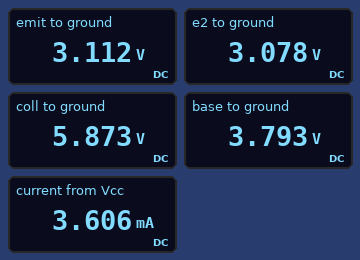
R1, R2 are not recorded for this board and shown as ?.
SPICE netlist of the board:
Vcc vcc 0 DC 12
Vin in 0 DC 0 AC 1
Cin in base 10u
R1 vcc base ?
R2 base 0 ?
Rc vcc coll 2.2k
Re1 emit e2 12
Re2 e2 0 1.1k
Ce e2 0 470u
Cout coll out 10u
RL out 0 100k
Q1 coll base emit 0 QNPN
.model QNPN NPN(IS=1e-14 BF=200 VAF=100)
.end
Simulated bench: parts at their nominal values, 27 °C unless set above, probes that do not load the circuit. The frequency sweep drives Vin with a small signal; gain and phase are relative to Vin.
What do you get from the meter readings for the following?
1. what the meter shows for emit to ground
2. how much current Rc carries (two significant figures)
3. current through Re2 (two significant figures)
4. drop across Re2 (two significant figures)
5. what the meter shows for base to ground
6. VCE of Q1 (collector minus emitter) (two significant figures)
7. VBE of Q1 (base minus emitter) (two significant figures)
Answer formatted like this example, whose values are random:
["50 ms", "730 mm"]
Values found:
["3.112 V", "2.8 mA", "2.8 mA", "3.1 V", "3.793 V", "2.8 V", "680 mV"]
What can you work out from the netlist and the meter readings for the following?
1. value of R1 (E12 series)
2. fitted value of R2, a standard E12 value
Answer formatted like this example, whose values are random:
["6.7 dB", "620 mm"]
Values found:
["10 kΩ", "4.7 kΩ"]
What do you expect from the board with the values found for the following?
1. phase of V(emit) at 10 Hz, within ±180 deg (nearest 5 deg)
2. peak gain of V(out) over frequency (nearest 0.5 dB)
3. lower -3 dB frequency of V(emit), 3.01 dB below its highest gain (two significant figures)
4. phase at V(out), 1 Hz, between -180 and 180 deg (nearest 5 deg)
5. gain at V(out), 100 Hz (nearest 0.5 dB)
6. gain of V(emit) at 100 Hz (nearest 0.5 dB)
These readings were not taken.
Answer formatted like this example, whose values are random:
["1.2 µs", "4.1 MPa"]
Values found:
["15 deg", "40.0 dB", "3.2 Hz", "-25 deg", "39.5 dB", "-5.0 dB"]
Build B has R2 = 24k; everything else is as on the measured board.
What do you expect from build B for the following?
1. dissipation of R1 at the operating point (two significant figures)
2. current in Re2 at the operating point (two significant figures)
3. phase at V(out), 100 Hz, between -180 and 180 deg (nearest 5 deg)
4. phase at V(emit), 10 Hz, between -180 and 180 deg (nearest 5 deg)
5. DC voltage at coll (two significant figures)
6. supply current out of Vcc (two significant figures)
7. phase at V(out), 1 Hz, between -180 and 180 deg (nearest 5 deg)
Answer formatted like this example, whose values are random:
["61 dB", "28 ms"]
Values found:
["4.8 mW", "3.9 mA", "-90 deg", "20 deg", "4.4 V", "4.1 mA", "30 deg"]
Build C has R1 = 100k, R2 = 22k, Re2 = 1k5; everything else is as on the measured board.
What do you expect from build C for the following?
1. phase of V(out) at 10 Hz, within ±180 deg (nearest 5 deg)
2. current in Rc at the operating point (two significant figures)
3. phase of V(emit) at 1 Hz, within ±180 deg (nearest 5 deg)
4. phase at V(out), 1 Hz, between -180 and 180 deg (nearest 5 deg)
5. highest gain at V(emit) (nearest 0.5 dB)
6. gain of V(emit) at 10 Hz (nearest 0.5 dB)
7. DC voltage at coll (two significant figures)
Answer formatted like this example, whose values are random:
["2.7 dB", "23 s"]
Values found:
["-130 deg", "940 µA", "35 deg", "-60 deg", "-2.5 dB", "-4.0 dB", "9.9 V"]
